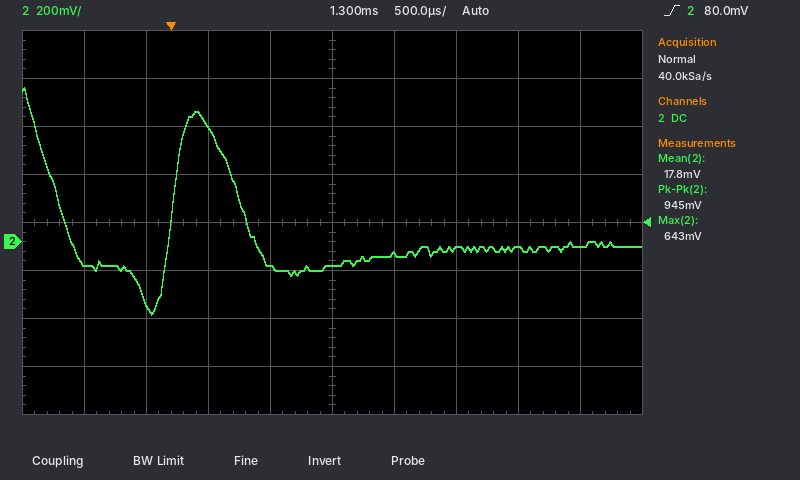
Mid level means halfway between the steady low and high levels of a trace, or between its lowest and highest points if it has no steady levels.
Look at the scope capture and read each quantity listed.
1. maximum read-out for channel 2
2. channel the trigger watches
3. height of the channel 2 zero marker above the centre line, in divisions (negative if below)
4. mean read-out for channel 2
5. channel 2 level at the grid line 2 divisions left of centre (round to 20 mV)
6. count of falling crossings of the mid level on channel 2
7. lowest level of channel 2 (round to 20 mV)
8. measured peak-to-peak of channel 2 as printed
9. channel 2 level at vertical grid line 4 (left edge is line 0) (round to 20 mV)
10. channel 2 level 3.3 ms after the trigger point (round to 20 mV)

643 mV
channel 2
-0.4 div
17.8 mV
480 mV
2
-300 mV
945 mV
-100 mV
-20 mV
